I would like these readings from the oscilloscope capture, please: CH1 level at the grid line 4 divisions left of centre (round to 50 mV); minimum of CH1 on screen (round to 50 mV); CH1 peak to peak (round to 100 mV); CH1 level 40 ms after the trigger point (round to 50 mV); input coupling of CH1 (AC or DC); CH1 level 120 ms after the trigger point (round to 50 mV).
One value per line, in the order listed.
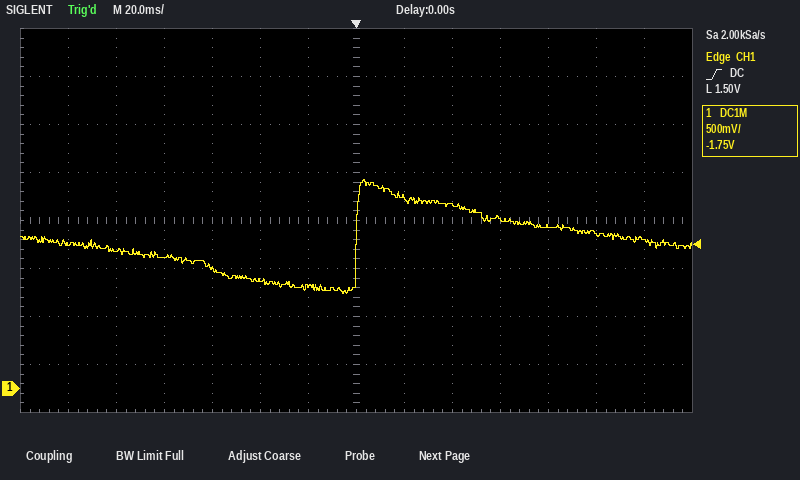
1.35 V
1.00 V
1.20 V
1.90 V
DC
1.55 V
